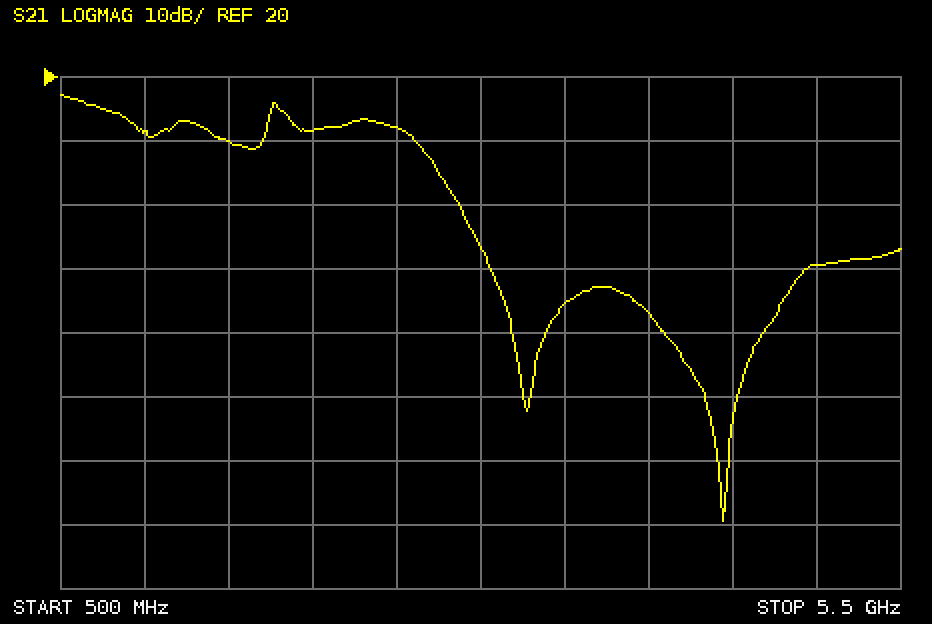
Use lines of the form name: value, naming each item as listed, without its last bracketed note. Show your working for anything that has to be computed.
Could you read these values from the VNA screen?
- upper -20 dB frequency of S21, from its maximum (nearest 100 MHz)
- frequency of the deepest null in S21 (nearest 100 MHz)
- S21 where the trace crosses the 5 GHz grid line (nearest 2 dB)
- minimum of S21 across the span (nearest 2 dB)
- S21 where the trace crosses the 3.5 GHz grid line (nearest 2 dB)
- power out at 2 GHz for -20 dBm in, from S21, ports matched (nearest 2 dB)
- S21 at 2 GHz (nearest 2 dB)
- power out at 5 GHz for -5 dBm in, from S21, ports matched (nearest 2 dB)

upper -20 dB frequency of S21, from its maximum: 2.9 GHz
frequency of the deepest null in S21: 4.4 GHz
S21 where the trace crosses the 5 GHz grid line: -10 dB
minimum of S21 across the span: -50 dB
S21 where the trace crosses the 3.5 GHz grid line: -16 dB
power out at 2 GHz for -20 dBm in, from S21, ports matched: -20 dBm + (12 dB) = -8 dBm
S21 at 2 GHz: 12 dB
power out at 5 GHz for -5 dBm in, from S21, ports matched: -5 dBm + (-10 dB) = -14 dBm
